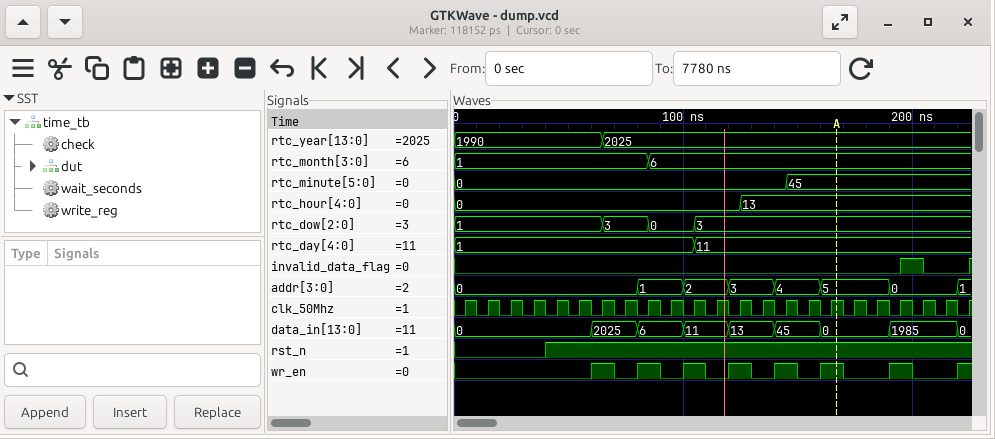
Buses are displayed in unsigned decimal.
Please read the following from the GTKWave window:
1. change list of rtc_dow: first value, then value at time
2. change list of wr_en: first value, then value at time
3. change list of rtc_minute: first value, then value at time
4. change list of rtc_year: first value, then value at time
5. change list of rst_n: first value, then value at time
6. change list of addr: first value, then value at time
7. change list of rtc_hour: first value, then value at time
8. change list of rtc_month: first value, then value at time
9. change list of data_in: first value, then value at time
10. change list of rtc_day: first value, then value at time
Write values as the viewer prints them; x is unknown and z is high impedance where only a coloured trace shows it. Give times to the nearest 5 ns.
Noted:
1, 3 at 65 ns, 0 at 85 ns, 3 at 105 ns
0, 1 at 60 ns, 0 at 70 ns, 1 at 80 ns, 0 at 90 ns, 1 at 100 ns, 0 at 110 ns, 1 at 120 ns, 0 at 130 ns, 1 at 140 ns, 0 at 150 ns, 1 at 160 ns, 0 at 170 ns, 1 at 190 ns, 0 at 200 ns, 1 at 220 ns
0, 45 at 145 ns
1990, 2025 at 65 ns
0, 1 at 40 ns
0, 1 at 80 ns, 2 at 100 ns, 3 at 120 ns, 4 at 140 ns, 5 at 160 ns, 0 at 190 ns, 1 at 220 ns
0, 13 at 125 ns
1, 6 at 85 ns
0, 2025 at 60 ns, 6 at 80 ns, 11 at 100 ns, 13 at 120 ns, 45 at 140 ns, 0 at 160 ns, 1985 at 190 ns, 0 at 220 ns
1, 11 at 105 ns
